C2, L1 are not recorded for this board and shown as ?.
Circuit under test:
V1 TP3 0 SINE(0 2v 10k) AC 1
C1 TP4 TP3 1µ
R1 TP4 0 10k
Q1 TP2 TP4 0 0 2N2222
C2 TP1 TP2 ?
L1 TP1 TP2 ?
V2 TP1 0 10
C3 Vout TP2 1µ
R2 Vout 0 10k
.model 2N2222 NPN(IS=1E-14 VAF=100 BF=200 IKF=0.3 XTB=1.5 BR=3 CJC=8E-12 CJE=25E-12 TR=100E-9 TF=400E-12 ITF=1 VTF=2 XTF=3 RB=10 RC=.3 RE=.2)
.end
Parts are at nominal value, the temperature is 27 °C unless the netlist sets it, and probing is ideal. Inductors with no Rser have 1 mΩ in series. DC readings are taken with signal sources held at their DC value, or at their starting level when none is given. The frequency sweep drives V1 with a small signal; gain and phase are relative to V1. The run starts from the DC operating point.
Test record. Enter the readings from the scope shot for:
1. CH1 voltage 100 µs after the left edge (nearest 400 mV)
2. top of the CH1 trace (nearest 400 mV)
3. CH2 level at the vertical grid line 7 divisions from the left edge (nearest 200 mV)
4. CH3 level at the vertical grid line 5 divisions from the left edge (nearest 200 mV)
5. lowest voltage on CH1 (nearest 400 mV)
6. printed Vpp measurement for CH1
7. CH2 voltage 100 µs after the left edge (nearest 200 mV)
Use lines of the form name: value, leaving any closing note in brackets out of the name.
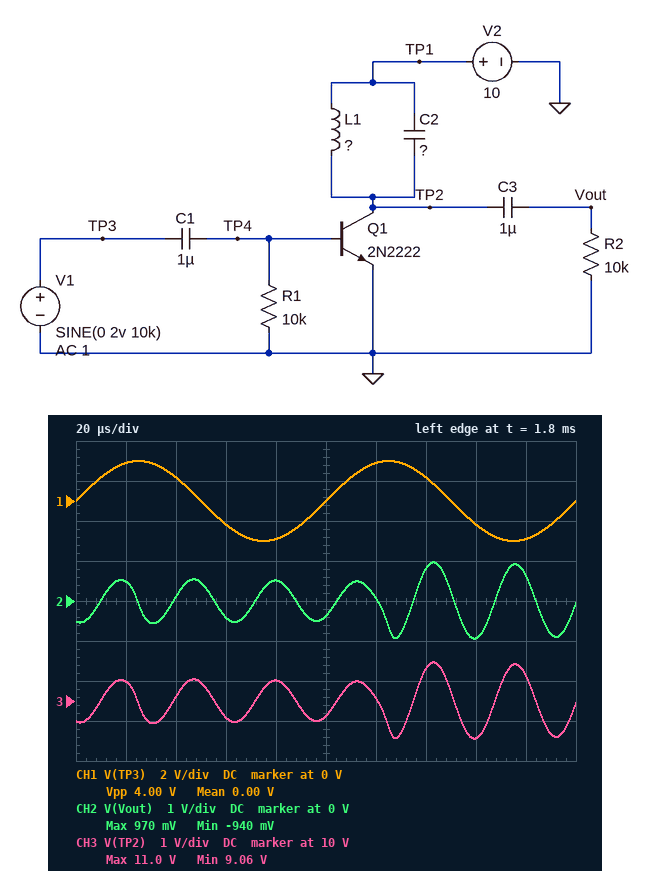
CH1 voltage 100 µs after the left edge: 0 V
top of the CH1 trace: 2.0 V
CH2 level at the vertical grid line 7 divisions from the left edge: 800 mV
CH3 level at the vertical grid line 5 divisions from the left edge: 9.6 V
lowest voltage on CH1: -2.0 V
printed Vpp measurement for CH1: 4.00 V
CH2 voltage 100 µs after the left edge: -400 mV
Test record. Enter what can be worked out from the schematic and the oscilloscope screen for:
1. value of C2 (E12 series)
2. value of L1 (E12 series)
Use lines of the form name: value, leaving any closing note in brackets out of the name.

value of C2: 33 nF
value of L1: 820 µH
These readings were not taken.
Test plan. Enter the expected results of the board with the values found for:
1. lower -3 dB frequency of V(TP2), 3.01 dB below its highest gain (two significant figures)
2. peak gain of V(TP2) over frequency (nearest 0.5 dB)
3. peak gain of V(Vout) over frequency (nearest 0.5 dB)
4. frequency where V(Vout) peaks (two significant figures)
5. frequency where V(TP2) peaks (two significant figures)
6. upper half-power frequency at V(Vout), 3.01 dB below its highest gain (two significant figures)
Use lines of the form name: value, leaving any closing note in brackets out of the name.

lower -3 dB frequency of V(TP2), 3.01 dB below its highest gain: 30 kHz
peak gain of V(TP2) over frequency: -44.0 dB
peak gain of V(Vout) over frequency: -44.0 dB
frequency where V(Vout) peaks: 31 kHz
frequency where V(TP2) peaks: 31 kHz
upper half-power frequency at V(Vout), 3.01 dB below its highest gain: 31 kHz
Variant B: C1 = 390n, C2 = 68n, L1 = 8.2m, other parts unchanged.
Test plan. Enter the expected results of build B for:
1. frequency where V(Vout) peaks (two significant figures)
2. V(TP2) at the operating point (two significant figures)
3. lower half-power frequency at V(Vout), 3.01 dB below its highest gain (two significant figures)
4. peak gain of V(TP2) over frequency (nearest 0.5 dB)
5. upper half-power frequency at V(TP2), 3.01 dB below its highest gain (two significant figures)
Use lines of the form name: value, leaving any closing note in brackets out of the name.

frequency where V(Vout) peaks: 6.7 kHz
V(TP2) at the operating point: 10 V
lower half-power frequency at V(Vout), 3.01 dB below its highest gain: 6.6 kHz
peak gain of V(TP2) over frequency: -57.0 dB
upper half-power frequency at V(TP2), 3.01 dB below its highest gain: 6.9 kHz
